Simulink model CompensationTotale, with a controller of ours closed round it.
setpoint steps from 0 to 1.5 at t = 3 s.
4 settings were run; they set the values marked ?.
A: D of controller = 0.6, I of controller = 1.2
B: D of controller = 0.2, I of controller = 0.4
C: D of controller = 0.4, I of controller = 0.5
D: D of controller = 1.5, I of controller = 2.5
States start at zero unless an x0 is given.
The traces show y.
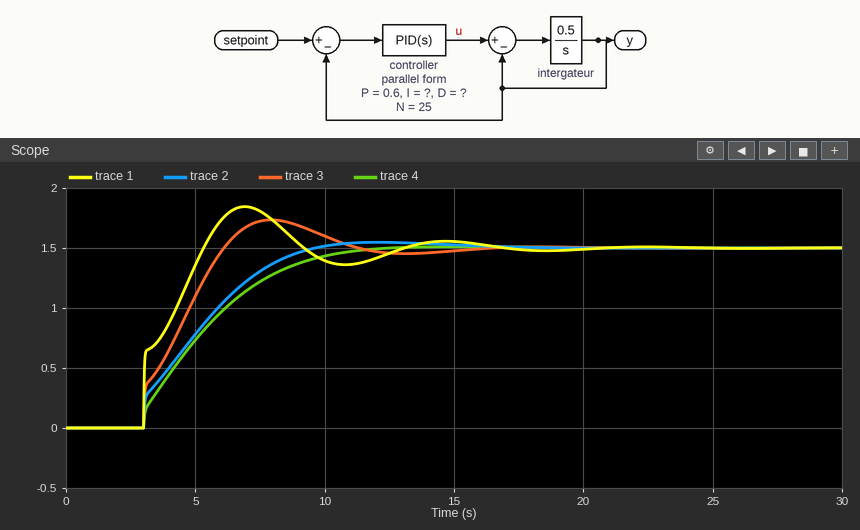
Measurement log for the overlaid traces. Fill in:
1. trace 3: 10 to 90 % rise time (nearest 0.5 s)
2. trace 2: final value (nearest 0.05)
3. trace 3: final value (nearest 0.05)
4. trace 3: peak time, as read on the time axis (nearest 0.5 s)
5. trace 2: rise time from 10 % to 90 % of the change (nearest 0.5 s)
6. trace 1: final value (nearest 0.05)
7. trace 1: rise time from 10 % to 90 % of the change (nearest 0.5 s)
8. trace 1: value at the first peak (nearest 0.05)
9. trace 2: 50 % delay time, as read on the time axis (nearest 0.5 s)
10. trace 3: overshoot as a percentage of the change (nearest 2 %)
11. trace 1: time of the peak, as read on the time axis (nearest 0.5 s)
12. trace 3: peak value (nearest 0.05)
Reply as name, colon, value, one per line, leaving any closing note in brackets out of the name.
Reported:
trace 3: 10 to 90 % rise time: 2.5 s
trace 2: final value: 1.50
trace 3: final value: 1.50
trace 3: peak time, as read on the time axis: 8.0 s
trace 2: rise time from 10 % to 90 % of the change: 5.0 s
trace 1: final value: 1.50
trace 1: rise time from 10 % to 90 % of the change: 2.0 s
trace 1: value at the first peak: 1.85
trace 2: 50 % delay time, as read on the time axis: 5.0 s
trace 3: overshoot as a percentage of the change: 16 %
trace 1: time of the peak, as read on the time axis: 7.0 s
trace 3: peak value: 1.75
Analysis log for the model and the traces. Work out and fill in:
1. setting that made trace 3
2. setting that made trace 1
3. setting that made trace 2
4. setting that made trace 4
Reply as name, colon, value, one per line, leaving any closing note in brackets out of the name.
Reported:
setting that made trace 3: A
setting that made trace 1: D
setting that made trace 2: C
setting that made trace 4: B
